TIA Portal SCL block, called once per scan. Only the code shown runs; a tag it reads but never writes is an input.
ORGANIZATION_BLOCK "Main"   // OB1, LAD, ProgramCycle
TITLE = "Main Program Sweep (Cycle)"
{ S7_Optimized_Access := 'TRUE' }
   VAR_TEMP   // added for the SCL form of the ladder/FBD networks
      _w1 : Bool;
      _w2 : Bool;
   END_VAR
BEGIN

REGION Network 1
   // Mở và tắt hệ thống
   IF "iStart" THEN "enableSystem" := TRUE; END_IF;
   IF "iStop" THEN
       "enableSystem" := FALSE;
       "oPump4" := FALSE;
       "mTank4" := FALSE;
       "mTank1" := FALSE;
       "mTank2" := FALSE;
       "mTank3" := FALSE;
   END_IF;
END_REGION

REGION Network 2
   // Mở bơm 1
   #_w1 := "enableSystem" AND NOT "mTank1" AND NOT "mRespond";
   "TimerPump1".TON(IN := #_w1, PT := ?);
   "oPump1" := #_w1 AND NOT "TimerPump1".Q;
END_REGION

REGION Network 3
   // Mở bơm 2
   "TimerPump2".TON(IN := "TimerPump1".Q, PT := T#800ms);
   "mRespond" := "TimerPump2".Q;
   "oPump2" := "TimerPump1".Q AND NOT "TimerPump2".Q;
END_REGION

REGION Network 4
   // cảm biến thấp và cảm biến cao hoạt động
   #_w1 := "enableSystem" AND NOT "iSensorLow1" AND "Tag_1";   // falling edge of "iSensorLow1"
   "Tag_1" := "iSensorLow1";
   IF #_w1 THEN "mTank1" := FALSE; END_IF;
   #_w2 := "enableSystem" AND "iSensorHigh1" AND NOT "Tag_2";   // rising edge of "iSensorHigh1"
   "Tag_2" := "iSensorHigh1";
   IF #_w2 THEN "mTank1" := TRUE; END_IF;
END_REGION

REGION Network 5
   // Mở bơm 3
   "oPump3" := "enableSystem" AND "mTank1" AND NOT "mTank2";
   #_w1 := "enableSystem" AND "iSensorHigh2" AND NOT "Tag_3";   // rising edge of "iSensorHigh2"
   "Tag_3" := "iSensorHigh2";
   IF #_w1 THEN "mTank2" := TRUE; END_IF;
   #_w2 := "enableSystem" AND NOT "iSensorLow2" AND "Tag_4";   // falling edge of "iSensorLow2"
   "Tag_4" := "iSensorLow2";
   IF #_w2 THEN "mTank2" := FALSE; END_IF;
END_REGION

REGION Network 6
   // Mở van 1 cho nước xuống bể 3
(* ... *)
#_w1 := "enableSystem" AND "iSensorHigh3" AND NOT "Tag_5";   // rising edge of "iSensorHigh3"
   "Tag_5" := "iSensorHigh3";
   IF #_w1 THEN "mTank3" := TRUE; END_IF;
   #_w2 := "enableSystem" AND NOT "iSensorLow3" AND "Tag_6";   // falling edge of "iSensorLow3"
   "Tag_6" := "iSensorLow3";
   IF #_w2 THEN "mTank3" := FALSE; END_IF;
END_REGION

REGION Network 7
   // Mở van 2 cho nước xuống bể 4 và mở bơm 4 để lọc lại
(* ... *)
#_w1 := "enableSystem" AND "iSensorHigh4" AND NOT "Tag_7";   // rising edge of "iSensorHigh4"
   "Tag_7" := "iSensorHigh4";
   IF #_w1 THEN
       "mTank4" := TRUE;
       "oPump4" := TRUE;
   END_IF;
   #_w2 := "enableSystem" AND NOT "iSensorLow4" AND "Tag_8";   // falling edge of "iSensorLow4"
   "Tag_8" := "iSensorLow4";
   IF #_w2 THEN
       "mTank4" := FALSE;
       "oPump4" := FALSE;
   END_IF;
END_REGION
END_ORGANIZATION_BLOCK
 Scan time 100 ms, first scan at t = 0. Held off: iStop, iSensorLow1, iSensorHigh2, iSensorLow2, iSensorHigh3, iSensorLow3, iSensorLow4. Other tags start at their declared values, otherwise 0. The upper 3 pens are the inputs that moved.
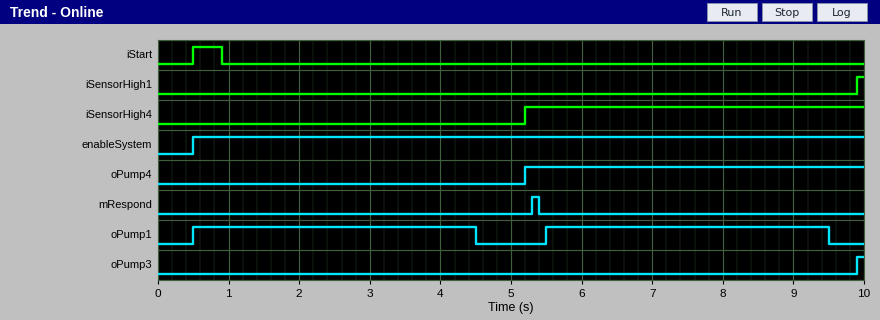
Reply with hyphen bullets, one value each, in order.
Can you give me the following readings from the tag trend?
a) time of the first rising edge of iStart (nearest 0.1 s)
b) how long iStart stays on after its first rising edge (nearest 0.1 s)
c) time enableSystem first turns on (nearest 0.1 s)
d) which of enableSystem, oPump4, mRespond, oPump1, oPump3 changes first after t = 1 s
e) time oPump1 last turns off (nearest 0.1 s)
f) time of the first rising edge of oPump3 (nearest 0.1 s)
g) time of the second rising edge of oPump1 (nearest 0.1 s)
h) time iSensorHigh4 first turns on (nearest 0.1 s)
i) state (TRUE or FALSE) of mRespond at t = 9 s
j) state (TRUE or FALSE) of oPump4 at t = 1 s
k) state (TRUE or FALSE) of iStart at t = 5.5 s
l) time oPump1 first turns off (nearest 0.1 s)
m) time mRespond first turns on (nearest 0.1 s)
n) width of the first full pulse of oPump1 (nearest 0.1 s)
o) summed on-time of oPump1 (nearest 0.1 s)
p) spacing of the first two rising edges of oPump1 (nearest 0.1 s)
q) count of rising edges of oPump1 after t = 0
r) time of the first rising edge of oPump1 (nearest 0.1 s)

- 0.5 s
- 0.4 s
- 0.5 s
- oPump1
- 9.5 s
- 9.9 s
- 5.5 s
- 5.2 s
- FALSE
- FALSE
- FALSE
- 4.5 s
- 5.3 s
- 4.0 s
- 8.0 s
- 5.0 s
- 2
- 0.5 s
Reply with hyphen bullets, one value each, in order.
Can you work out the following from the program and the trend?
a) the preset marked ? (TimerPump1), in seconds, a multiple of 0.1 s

- 4.0 s
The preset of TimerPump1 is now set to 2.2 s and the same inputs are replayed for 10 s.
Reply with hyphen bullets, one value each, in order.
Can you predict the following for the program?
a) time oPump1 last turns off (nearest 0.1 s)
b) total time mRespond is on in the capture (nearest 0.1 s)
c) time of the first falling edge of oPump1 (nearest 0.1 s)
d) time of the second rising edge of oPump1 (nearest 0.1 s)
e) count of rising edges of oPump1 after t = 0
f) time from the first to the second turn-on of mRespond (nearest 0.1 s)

- 9.1 s
- 0.3 s
- 2.7 s
- 3.7 s
- 3
- 3.2 s
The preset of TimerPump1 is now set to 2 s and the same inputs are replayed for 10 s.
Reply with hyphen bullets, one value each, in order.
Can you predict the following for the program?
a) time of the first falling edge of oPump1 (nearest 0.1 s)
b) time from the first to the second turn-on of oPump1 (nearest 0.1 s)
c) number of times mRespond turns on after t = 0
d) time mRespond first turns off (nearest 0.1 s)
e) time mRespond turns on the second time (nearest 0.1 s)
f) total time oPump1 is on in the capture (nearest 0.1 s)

- 2.5 s
- 3.0 s
- 3
- 3.4 s
- 6.3 s
- 6.5 s
